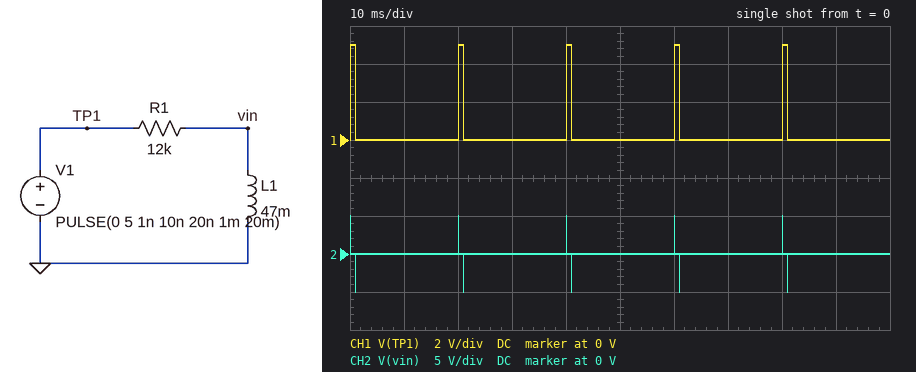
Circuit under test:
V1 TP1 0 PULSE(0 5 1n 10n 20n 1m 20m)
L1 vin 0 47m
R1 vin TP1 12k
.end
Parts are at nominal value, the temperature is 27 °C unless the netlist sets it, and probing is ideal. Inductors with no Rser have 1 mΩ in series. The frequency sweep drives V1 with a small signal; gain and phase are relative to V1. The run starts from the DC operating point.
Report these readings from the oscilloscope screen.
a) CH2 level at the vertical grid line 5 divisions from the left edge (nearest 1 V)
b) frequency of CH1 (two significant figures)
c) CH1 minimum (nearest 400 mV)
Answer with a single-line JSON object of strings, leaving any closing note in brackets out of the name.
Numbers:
{"CH2 level at the vertical grid line 5 divisions from the left edge": "0 V", "frequency of CH1": "50 Hz", "CH1 minimum": "0 V"}
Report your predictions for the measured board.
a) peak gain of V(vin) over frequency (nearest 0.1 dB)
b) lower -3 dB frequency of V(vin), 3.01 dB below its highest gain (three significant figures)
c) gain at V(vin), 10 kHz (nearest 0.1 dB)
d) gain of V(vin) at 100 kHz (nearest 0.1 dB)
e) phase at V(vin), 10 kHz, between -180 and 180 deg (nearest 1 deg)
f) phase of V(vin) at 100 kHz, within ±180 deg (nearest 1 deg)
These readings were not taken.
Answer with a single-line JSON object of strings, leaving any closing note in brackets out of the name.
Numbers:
{"peak gain of V(vin) over frequency": "0 dB", "lower -3 dB frequency of V(vin), 3.01 dB below its highest gain": "40.6 kHz", "gain at V(vin), 10 kHz": "-12.4 dB", "gain of V(vin) at 100 kHz": "-0.7 dB", "phase at V(vin), 10 kHz, between -180 and 180 deg": "76 deg", "phase of V(vin) at 100 kHz, within ±180 deg": "22 deg"}
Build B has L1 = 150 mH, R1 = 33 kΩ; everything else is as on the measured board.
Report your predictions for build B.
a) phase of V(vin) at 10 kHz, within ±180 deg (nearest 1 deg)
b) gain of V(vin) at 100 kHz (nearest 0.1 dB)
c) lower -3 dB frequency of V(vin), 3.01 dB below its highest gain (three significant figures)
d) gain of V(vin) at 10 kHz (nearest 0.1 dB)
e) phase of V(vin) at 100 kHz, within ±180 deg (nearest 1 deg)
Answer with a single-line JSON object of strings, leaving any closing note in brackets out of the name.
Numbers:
{"phase of V(vin) at 10 kHz, within ±180 deg": "74 deg", "gain of V(vin) at 100 kHz": "-0.5 dB", "lower -3 dB frequency of V(vin), 3.01 dB below its highest gain": "35.0 kHz", "gain of V(vin) at 10 kHz": "-11.2 dB", "phase of V(vin) at 100 kHz, within ±180 deg": "19 deg"}
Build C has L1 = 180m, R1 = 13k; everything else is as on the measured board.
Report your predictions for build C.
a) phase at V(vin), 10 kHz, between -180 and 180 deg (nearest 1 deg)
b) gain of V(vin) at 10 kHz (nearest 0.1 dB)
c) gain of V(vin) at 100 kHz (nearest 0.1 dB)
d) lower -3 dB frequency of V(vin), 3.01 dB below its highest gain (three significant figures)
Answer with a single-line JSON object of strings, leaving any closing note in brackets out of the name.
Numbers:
{"phase at V(vin), 10 kHz, between -180 and 180 deg": "49 deg", "gain of V(vin) at 10 kHz": "-3.7 dB", "gain of V(vin) at 100 kHz": "-0.1 dB", "lower -3 dB frequency of V(vin), 3.01 dB below its highest gain": "11.5 kHz"}
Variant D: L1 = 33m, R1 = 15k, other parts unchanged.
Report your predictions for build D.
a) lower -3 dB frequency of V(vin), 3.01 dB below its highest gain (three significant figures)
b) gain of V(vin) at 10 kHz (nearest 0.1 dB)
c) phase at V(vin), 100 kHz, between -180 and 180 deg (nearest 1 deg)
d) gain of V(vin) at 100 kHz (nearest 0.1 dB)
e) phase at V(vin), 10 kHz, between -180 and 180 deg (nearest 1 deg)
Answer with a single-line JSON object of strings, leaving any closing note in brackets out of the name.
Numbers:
{"lower -3 dB frequency of V(vin), 3.01 dB below its highest gain": "72.3 kHz", "gain of V(vin) at 10 kHz": "-17.3 dB", "phase at V(vin), 100 kHz, between -180 and 180 deg": "36 deg", "gain of V(vin) at 100 kHz": "-1.8 dB", "phase at V(vin), 10 kHz, between -180 and 180 deg": "82 deg"}
